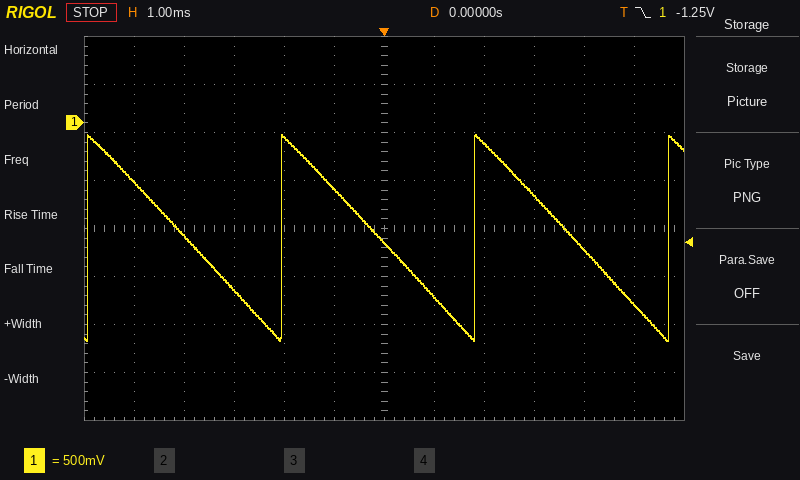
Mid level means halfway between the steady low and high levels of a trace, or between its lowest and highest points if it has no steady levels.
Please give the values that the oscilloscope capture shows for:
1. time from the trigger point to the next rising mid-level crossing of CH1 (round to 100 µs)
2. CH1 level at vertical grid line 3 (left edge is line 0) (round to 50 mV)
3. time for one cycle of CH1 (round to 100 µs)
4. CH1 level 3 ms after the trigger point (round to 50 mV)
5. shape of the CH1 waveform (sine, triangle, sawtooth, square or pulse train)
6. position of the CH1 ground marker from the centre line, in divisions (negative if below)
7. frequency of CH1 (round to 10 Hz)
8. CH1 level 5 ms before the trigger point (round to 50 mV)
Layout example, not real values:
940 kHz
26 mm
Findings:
1.8 ms
-1.75 V
3.9 ms
-750 mV
sawtooth
+2.2 div
260 Hz
-600 mV
